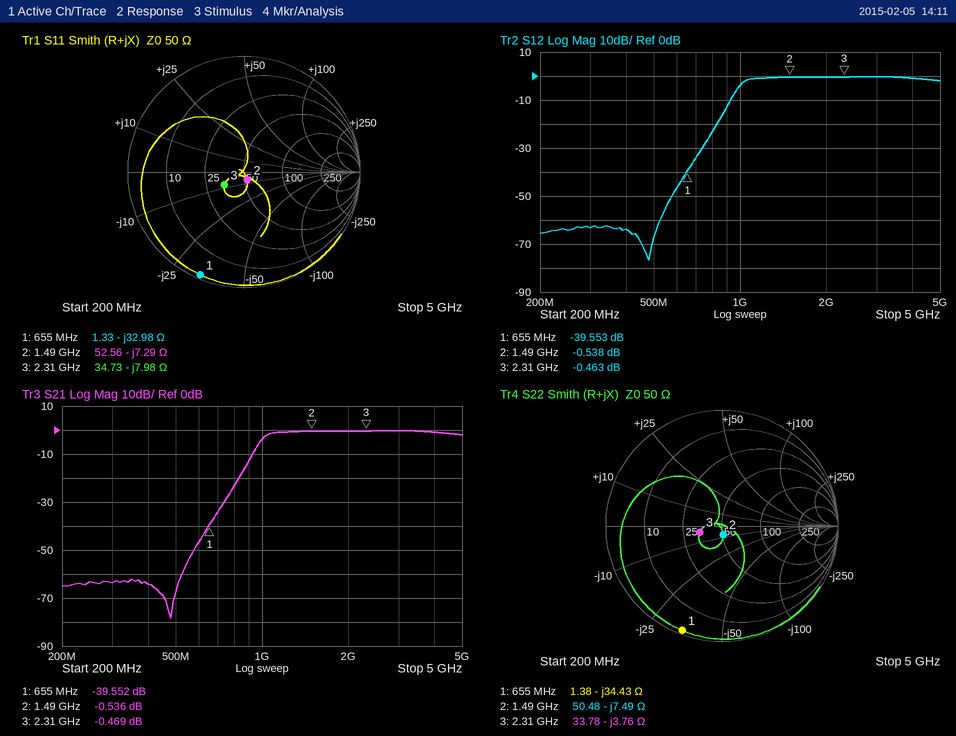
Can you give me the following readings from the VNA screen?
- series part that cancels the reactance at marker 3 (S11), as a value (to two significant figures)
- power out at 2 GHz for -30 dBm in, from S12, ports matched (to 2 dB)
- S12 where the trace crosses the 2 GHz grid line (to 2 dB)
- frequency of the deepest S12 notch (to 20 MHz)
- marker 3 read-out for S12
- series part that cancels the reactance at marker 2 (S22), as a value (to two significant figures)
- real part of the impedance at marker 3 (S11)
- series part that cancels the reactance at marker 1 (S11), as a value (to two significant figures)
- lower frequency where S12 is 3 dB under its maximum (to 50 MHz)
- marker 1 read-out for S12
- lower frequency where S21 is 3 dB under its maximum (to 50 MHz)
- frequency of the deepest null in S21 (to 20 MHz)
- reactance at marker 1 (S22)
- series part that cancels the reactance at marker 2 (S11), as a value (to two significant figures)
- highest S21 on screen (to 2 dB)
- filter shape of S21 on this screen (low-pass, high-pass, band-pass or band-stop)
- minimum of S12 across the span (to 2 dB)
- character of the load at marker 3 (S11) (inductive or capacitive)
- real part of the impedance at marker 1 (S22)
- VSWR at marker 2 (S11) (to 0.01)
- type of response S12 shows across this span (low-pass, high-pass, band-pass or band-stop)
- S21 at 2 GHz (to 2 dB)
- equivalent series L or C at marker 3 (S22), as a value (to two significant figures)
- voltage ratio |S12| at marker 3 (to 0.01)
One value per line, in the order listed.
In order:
550 pH
-30 dBm
0 dB
480 MHz
-0.463 dB
800 pH
34.73 Ω
8.0 nH
1.00 GHz
-39.553 dB
1.00 GHz
480 MHz
-34.43 Ω
780 pH
0 dB
high-pass
-76 dB
capacitive
1.38 Ω
1.16
high-pass
0 dB
18 pF
0.95
